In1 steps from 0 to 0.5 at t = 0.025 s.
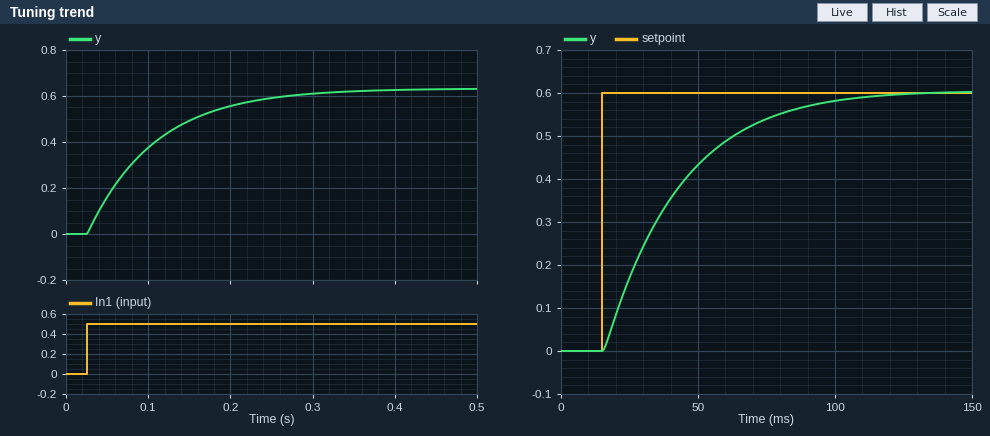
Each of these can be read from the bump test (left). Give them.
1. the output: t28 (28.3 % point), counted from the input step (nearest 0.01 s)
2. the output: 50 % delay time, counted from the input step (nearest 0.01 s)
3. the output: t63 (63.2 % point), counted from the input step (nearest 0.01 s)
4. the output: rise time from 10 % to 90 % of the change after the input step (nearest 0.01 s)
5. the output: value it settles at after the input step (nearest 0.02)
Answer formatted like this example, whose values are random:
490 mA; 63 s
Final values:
0.03 s; 0.06 s; 0.08 s; 0.18 s; 0.64
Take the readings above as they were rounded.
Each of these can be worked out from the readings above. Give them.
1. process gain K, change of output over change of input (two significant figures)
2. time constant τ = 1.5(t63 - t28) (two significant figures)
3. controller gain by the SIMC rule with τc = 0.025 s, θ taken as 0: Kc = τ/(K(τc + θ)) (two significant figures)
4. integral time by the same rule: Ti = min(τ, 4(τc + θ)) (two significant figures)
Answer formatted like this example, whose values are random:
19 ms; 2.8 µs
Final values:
1.3; 0.075 s; 2.3; 0.075 s
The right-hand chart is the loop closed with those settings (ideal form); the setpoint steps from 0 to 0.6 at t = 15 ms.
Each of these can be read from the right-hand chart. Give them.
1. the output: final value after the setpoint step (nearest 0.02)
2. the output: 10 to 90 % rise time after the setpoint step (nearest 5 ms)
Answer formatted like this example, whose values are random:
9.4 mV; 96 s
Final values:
0.60; 55 ms
